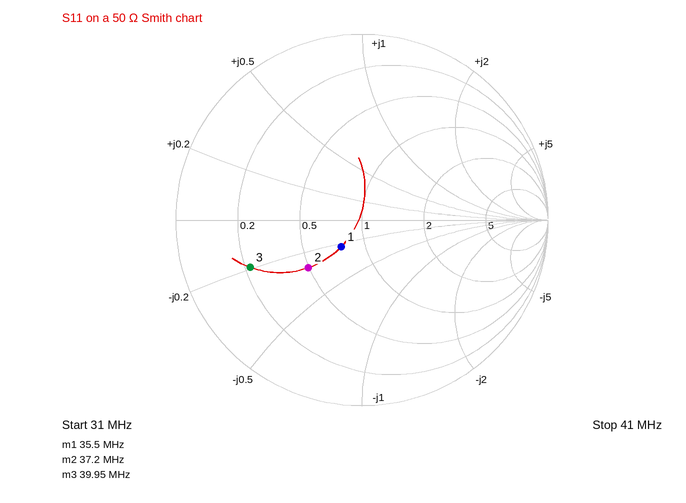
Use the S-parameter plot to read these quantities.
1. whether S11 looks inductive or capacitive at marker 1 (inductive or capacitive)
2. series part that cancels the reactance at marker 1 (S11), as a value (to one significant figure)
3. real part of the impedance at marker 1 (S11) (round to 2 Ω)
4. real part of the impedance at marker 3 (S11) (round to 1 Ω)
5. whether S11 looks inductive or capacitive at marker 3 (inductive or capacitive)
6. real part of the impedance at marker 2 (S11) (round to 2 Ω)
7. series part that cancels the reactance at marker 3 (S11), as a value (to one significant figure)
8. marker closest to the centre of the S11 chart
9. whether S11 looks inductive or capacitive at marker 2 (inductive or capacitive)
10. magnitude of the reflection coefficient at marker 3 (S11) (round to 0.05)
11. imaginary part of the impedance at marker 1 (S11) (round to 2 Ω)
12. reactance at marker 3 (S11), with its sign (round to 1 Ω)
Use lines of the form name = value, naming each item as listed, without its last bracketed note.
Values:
whether S11 looks inductive or capacitive at marker 1 = capacitive
series part that cancels the reactance at marker 1 (S11), as a value = 50 nH
real part of the impedance at marker 1 (S11) = 38 Ω
real part of the impedance at marker 3 (S11) = 11 Ω
whether S11 looks inductive or capacitive at marker 3 = capacitive
real part of the impedance at marker 2 (S11) = 24 Ω
series part that cancels the reactance at marker 3 (S11), as a value = 40 nH
marker closest to the centre of the S11 chart = marker 1
whether S11 looks inductive or capacitive at marker 2 = capacitive
magnitude of the reflection coefficient at marker 3 (S11) = 0.65
imaginary part of the impedance at marker 1 (S11) = -12 Ω
reactance at marker 3 (S11), with its sign = -10 Ω
